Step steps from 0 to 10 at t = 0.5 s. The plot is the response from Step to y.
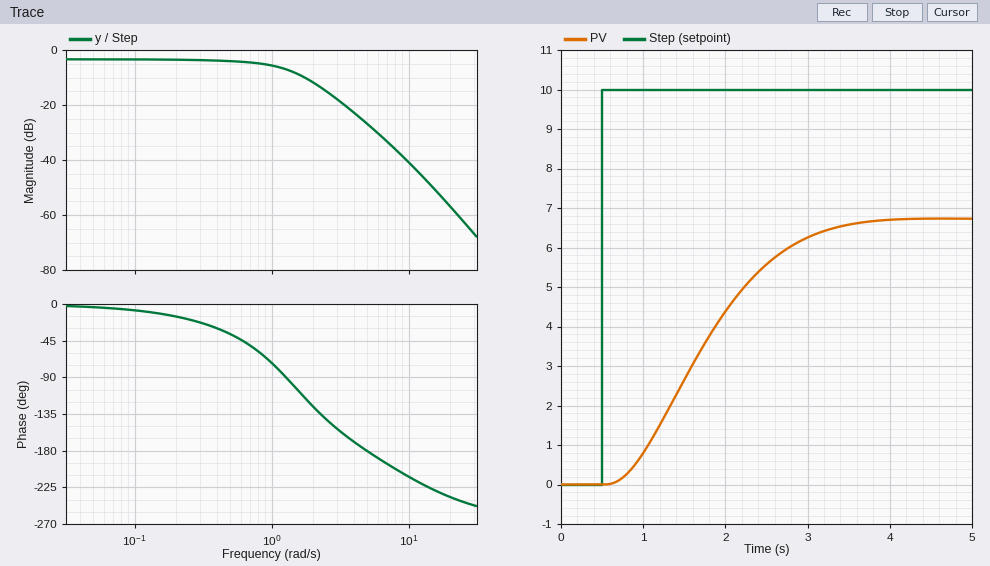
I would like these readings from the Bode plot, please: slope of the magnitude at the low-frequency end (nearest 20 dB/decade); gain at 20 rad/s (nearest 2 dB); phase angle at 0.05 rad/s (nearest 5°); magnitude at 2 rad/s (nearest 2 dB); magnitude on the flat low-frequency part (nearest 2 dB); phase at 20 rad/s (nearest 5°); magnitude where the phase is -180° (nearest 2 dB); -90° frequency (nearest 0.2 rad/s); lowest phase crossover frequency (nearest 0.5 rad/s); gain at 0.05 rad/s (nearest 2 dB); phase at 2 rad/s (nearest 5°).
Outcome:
0 dB/decade
-56 dB
-5°
-12 dB
-4 dB
-235°
-26 dB
1.2 rad/s
5.0 rad/s
-4 dB
-125°
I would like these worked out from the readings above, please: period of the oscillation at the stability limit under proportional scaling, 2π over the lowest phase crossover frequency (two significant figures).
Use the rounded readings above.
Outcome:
1.3 s
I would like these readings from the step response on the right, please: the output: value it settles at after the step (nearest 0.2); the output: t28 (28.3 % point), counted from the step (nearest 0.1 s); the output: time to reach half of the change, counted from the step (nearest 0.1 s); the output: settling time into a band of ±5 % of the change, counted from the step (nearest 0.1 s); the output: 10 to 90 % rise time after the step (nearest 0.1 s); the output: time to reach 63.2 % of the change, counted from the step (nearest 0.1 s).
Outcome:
6.8
0.8 s
1.2 s
2.7 s
1.9 s
1.5 s
